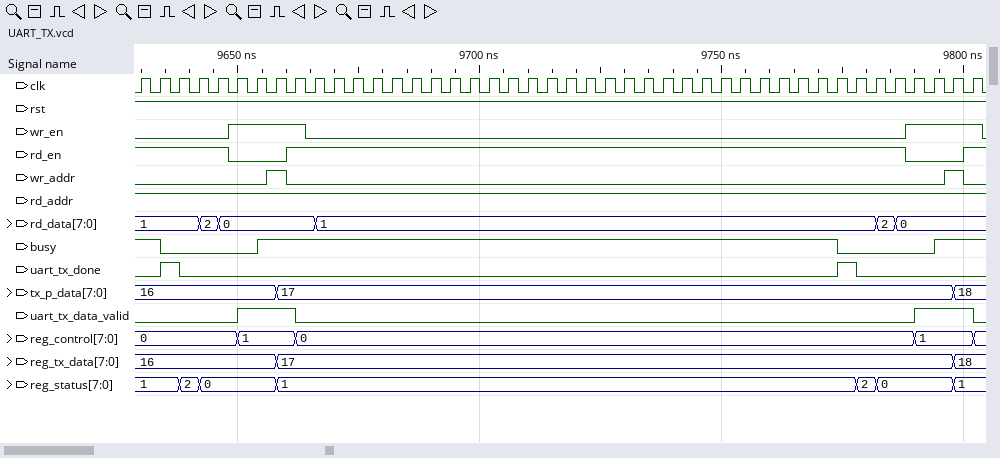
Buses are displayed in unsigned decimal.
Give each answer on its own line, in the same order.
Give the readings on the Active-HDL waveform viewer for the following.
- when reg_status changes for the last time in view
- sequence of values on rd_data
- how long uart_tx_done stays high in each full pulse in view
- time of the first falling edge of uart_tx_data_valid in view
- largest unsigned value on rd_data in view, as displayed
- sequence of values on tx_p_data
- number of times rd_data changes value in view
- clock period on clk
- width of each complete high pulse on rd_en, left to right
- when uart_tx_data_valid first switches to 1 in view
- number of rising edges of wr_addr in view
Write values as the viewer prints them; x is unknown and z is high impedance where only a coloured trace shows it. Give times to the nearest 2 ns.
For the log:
9798 ns
1, 2, 0, 1, 2, 0
4 ns, 4 ns
9662 ns
2
16, 17, 18
5
4 ns
128 ns
9650 ns
2
